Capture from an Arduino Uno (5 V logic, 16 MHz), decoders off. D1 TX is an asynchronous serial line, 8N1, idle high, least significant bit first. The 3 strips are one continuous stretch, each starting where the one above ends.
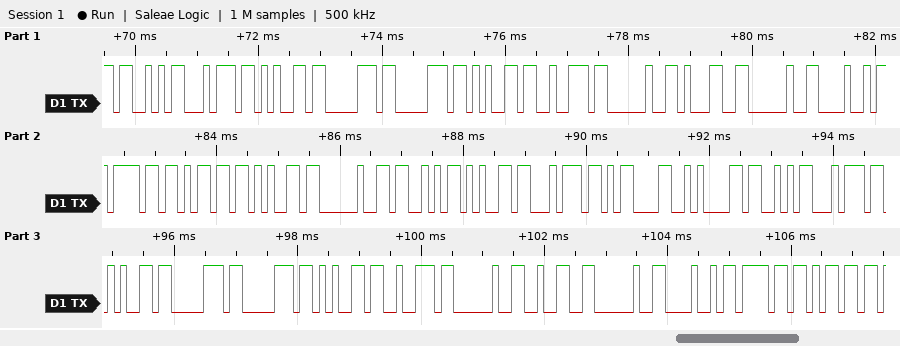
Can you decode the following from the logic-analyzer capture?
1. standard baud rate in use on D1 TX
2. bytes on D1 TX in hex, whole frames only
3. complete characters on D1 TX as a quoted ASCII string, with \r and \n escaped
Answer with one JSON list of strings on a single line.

["9600 baud", "0x53 0x74 0x65 0x70 0x70 0x65 0x72 0x20 0x31 0x20 0x48 0x6F 0x6D 0x65 0x20 0x53 0x65 0x74 0x0D 0x0A 0x53 0x74 0x65 0x70 0x70 0x65 0x72 0x20 0x32 0x20 0x48 0x6F 0x6D", "\"Stepper 1 Home Set\\r\\nStepper 2 Hom\""]
